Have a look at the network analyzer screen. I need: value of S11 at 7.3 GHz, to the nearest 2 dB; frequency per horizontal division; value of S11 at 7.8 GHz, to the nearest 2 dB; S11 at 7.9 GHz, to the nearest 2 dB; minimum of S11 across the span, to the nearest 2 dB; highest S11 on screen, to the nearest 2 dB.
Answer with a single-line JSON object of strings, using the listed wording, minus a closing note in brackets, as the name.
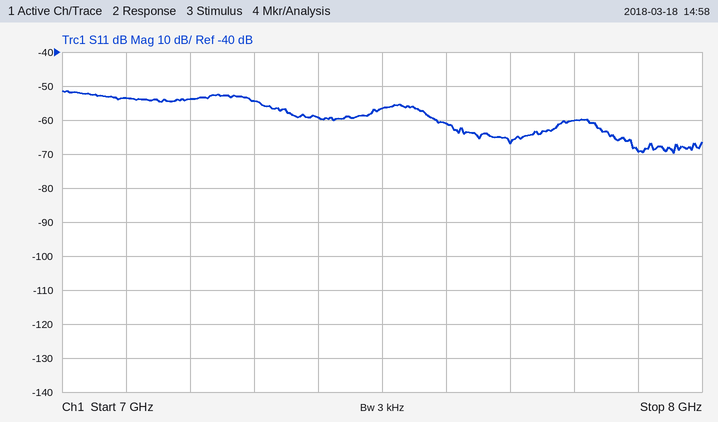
{"value of S11 at 7.3 GHz, to the nearest 2 dB": "-54 dB", "frequency per horizontal division": "100 MHz", "value of S11 at 7.8 GHz, to the nearest 2 dB": "-60 dB", "S11 at 7.9 GHz, to the nearest 2 dB": "-70 dB", "minimum of S11 across the span, to the nearest 2 dB": "-70 dB", "highest S11 on screen, to the nearest 2 dB": "-52 dB"}
